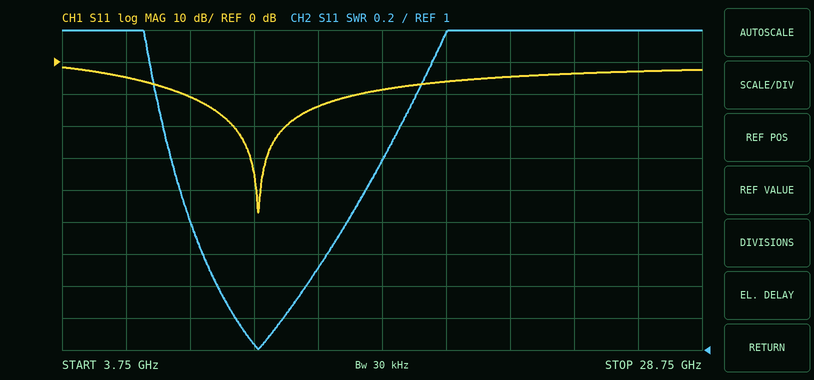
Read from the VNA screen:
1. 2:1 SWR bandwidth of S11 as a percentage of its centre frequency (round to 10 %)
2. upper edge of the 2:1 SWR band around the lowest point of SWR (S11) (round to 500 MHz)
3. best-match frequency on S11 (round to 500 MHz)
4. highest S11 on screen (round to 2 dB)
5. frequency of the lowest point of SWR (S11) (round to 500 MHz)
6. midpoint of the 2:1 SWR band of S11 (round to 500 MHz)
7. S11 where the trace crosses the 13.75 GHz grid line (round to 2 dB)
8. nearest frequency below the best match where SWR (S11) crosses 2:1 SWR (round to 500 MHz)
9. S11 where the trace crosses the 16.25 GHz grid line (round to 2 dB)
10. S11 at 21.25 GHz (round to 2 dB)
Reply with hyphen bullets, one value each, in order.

- 60 %
- 15.5 GHz
- 11.5 GHz
- -2 dB
- 11.5 GHz
- 12.0 GHz
- -14 dB
- 8.5 GHz
- -8 dB
- -4 dB
